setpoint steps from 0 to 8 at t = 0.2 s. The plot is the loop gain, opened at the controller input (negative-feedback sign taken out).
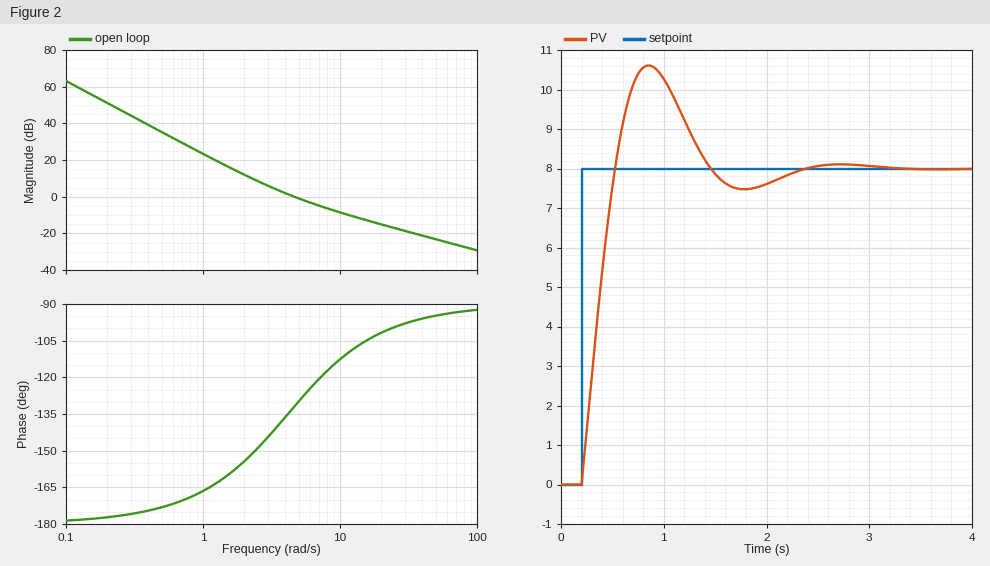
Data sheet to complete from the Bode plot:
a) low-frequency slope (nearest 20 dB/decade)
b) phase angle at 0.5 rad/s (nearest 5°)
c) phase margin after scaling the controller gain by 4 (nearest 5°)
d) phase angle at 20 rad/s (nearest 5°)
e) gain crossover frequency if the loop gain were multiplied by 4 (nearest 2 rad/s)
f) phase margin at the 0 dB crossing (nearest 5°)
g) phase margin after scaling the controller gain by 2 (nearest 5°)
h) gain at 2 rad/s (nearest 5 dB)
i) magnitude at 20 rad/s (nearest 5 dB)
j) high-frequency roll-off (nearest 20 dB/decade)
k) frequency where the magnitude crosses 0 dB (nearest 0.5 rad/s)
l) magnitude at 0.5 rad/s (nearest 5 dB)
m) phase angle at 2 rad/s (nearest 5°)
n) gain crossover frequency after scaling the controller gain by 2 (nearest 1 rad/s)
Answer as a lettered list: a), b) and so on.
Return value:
a) -40 dB/decade
b) -175°
c) 75°
d) -100°
e) 14 rad/s
f) 50°
g) 60°
h) 10 dB
i) -15 dB
j) -20 dB/decade
k) 4.5 rad/s
l) 35 dB
m) -155°
n) 8 rad/s
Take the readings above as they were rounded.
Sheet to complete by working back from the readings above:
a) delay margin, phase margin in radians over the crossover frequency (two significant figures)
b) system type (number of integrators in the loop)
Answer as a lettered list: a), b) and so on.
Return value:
a) 0.19 s
b) 2
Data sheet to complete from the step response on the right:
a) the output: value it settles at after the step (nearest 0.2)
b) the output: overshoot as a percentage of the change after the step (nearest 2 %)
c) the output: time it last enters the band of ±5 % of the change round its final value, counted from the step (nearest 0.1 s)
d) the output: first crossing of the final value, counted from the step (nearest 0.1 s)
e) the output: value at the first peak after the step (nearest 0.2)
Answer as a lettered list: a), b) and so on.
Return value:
a) 8.0
b) 32 %
c) 1.8 s
d) 0.3 s
e) 10.6
